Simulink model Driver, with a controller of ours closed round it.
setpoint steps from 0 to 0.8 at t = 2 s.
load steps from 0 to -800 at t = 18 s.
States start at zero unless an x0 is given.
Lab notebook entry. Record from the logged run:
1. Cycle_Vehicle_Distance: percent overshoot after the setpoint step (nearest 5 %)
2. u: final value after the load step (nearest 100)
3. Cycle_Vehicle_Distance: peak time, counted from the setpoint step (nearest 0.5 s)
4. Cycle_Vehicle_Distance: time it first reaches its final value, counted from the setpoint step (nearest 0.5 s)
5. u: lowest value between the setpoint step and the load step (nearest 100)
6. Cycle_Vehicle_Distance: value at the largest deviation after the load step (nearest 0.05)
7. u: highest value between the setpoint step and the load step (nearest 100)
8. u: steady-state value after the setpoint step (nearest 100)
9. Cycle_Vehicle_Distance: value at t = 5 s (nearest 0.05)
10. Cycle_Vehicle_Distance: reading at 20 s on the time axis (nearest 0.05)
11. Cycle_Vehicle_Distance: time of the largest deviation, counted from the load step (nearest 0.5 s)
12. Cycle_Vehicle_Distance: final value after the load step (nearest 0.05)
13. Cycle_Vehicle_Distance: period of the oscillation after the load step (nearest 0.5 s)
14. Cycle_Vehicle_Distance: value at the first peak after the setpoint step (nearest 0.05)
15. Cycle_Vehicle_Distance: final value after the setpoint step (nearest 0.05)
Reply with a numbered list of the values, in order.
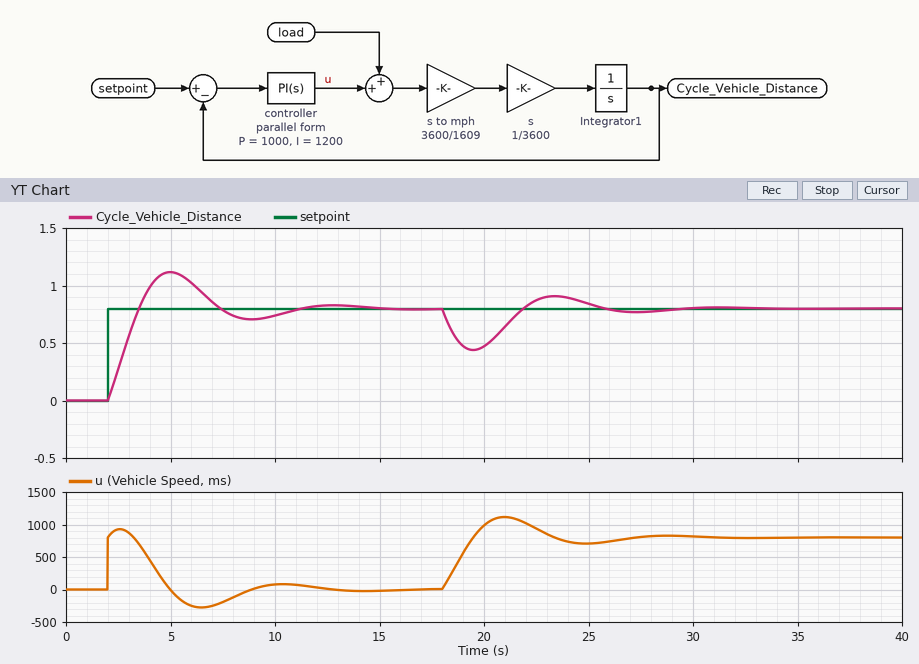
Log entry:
1. 40 %
2. 800
3. 3.0 s
4. 1.5 s
5. -300
6. 0.45
7. 900
8. 0
9. 1.10
10. 0.45
11. 1.5 s
12. 0.80
13. 8.0 s
14. 1.10
15. 0.80
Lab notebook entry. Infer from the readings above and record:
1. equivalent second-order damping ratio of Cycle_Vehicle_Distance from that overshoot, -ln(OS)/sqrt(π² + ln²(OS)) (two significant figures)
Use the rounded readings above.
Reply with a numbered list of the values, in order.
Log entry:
1. 0.28
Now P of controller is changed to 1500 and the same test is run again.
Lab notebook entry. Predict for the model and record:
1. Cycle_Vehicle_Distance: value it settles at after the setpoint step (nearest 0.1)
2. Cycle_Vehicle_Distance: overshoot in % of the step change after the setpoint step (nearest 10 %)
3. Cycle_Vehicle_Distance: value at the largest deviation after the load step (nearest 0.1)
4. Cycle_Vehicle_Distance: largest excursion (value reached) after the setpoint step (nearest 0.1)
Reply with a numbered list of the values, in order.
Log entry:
1. 0.8
2. 30 %
3. 0.5
4. 1.0
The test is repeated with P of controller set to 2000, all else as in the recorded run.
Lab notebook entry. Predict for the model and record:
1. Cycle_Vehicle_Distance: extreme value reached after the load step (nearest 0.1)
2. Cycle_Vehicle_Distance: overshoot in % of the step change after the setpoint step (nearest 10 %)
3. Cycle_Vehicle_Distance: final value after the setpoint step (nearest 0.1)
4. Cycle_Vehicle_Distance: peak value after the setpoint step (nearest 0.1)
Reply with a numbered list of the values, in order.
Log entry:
1. 0.5
2. 20 %
3. 0.8
4. 1.0
